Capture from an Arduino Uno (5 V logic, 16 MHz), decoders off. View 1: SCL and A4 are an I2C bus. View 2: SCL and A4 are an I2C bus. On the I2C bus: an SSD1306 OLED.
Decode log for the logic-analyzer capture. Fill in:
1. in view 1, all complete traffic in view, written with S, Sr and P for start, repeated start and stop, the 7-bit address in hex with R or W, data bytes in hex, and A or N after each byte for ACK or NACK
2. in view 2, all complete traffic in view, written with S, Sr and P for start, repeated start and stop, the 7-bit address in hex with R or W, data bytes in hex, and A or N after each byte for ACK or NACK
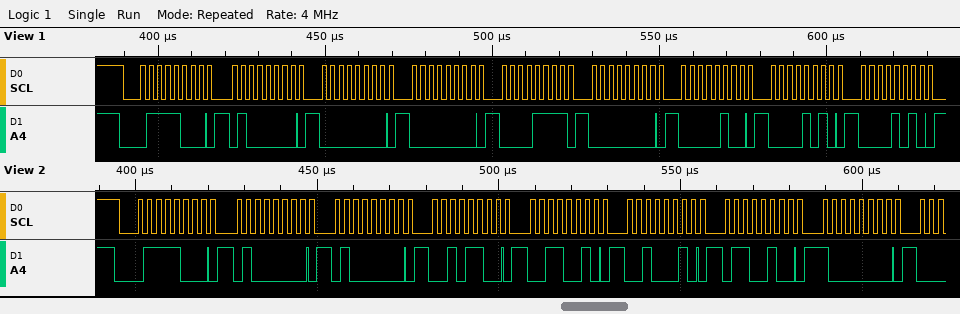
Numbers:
S 3CW A 40 A 00 A 00 A 0F A 00 A 04 A 0A A 0A A
S 3CW A 40 A 40 A 2C A 32 A 22 A 64 A 80 A
